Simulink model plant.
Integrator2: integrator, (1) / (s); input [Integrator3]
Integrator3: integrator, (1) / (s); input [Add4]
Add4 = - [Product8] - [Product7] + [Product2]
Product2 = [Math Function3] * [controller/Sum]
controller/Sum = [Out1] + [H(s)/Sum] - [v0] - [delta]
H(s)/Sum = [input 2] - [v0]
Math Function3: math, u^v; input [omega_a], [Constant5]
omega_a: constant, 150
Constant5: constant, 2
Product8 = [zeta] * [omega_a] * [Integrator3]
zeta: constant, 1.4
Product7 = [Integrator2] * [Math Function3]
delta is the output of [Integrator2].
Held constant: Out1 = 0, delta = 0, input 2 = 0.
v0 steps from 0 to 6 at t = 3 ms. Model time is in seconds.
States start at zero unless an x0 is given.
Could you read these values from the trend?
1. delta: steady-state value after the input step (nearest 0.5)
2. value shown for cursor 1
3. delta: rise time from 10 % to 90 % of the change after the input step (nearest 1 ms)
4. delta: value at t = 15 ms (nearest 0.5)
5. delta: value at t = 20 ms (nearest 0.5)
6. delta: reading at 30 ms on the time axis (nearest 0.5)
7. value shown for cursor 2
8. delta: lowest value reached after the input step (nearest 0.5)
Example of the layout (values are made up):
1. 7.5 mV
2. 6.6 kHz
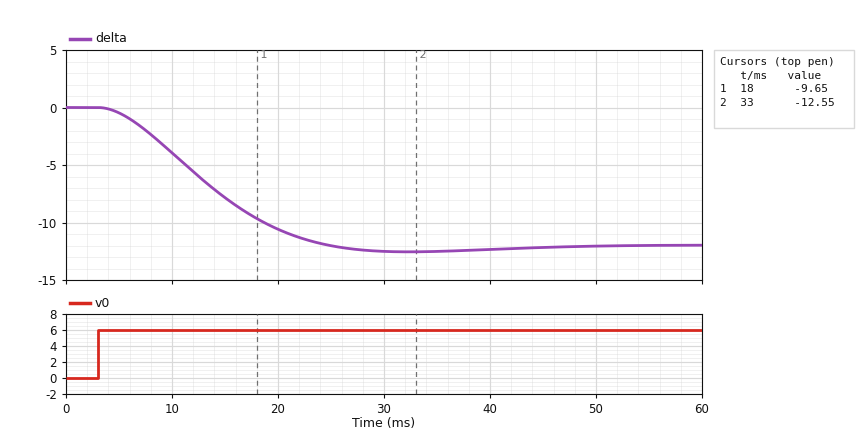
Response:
1. -12.0
2. -9.65
3. 14 ms
4. -8.0
5. -10.5
6. -12.5
7. -12.55
8. -12.5
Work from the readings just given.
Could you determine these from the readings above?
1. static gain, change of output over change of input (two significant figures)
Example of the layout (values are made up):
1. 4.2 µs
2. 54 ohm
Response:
1. -2.0
